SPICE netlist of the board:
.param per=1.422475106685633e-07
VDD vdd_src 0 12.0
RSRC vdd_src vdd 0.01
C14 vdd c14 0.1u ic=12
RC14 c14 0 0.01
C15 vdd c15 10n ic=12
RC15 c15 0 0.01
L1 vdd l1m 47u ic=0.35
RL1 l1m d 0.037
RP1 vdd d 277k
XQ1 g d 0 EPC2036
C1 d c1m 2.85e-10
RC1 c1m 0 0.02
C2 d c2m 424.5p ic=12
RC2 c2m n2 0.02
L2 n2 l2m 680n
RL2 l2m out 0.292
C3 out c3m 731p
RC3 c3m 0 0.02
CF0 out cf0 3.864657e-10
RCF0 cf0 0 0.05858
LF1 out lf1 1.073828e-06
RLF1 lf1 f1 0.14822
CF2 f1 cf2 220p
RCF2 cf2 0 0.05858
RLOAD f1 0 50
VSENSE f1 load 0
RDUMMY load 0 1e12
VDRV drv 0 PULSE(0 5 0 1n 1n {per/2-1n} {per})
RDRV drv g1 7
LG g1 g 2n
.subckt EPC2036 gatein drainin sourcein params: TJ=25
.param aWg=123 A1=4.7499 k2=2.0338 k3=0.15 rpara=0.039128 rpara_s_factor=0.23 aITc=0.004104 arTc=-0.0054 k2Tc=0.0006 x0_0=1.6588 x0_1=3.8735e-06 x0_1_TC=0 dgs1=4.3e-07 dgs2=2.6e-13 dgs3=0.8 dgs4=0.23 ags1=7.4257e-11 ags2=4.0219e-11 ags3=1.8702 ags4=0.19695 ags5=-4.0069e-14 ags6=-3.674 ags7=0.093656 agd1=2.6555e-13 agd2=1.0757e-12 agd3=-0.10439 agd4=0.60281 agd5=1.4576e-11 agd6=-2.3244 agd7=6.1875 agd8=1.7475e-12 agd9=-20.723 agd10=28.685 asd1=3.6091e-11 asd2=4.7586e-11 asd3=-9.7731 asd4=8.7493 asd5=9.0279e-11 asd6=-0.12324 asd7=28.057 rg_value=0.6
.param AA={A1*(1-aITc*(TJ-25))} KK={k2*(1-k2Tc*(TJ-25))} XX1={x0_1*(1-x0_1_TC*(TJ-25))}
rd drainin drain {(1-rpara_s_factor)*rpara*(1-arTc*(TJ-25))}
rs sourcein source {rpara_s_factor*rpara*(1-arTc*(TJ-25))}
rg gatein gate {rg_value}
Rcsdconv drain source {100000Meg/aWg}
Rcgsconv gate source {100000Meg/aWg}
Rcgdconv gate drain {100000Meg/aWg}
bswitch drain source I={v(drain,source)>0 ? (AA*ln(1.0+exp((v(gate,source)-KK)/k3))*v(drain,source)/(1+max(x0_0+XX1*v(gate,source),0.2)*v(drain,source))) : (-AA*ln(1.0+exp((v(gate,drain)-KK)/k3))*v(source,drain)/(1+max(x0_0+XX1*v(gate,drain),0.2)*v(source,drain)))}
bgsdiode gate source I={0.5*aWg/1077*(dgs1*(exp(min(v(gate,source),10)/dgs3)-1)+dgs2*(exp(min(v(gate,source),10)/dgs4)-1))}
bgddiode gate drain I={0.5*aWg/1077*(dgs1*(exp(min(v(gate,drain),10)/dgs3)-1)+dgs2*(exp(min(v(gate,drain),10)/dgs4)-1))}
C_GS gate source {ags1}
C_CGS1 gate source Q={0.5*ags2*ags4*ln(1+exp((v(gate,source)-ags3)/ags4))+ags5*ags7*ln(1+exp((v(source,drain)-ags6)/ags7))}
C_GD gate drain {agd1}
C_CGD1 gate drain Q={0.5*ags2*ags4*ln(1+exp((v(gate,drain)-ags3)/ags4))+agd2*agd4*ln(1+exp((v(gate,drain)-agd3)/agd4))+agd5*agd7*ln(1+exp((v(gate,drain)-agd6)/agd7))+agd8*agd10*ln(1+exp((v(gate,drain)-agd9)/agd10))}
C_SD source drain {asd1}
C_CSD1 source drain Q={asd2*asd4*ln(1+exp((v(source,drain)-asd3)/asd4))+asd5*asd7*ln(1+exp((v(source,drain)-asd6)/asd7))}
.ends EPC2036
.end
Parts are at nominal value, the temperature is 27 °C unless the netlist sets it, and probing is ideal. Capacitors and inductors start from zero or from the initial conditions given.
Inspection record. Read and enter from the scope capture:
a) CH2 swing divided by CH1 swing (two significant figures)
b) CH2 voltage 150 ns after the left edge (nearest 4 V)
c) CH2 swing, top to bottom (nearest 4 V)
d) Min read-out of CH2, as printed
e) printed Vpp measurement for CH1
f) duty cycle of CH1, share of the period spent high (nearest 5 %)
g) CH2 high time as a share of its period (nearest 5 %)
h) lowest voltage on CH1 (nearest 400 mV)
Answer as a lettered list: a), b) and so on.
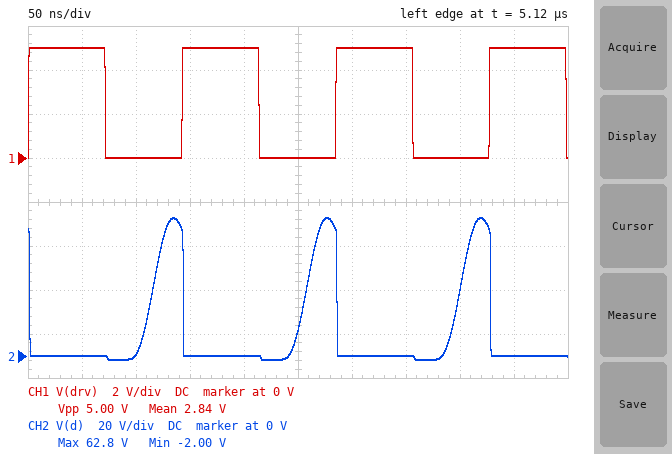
a) 13
b) 0 V
c) 64 V
d) -2.00 V
e) 5.00 V
f) 50 %
g) 20 %
h) 0 V
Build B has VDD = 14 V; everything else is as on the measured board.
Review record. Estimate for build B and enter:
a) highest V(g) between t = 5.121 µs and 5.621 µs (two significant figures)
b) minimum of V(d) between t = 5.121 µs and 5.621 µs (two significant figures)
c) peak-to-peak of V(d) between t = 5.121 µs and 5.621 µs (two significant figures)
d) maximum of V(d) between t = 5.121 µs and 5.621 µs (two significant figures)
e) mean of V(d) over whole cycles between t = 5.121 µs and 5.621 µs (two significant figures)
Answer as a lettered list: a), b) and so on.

a) 5.0 V
b) -2.0 V
c) 75 V
d) 73 V
e) 14 V
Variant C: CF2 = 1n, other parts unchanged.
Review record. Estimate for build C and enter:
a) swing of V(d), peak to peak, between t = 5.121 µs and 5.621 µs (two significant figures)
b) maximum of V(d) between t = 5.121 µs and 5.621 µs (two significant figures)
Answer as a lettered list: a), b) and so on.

a) 61 V
b) 59 V
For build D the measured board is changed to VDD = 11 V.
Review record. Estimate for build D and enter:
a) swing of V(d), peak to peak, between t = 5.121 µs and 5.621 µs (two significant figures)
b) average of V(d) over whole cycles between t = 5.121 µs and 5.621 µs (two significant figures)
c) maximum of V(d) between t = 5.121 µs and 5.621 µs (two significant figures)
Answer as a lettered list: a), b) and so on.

a) 60 V
b) 11 V
c) 58 V
